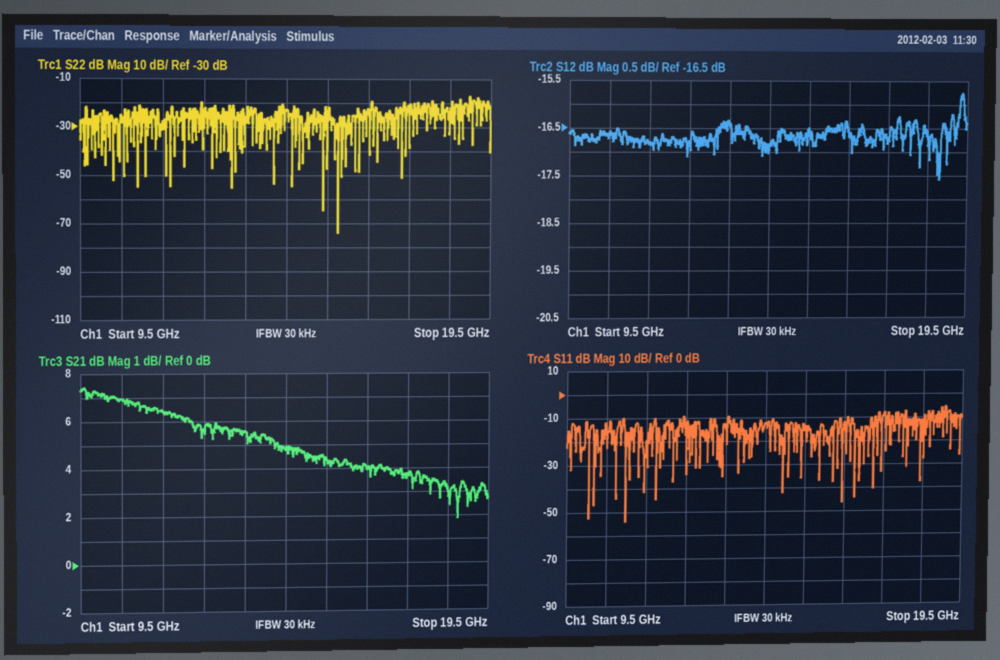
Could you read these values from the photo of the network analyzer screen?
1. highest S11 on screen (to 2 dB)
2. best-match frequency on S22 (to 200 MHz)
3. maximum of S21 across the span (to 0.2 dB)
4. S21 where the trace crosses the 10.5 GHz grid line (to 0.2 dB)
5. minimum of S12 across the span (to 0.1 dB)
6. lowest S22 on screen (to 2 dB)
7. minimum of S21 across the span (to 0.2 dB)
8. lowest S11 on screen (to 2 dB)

-6 dB
15.8 GHz
7.4 dB
7.0 dB
-17.6 dB
-74 dB
1.8 dB
-54 dB
